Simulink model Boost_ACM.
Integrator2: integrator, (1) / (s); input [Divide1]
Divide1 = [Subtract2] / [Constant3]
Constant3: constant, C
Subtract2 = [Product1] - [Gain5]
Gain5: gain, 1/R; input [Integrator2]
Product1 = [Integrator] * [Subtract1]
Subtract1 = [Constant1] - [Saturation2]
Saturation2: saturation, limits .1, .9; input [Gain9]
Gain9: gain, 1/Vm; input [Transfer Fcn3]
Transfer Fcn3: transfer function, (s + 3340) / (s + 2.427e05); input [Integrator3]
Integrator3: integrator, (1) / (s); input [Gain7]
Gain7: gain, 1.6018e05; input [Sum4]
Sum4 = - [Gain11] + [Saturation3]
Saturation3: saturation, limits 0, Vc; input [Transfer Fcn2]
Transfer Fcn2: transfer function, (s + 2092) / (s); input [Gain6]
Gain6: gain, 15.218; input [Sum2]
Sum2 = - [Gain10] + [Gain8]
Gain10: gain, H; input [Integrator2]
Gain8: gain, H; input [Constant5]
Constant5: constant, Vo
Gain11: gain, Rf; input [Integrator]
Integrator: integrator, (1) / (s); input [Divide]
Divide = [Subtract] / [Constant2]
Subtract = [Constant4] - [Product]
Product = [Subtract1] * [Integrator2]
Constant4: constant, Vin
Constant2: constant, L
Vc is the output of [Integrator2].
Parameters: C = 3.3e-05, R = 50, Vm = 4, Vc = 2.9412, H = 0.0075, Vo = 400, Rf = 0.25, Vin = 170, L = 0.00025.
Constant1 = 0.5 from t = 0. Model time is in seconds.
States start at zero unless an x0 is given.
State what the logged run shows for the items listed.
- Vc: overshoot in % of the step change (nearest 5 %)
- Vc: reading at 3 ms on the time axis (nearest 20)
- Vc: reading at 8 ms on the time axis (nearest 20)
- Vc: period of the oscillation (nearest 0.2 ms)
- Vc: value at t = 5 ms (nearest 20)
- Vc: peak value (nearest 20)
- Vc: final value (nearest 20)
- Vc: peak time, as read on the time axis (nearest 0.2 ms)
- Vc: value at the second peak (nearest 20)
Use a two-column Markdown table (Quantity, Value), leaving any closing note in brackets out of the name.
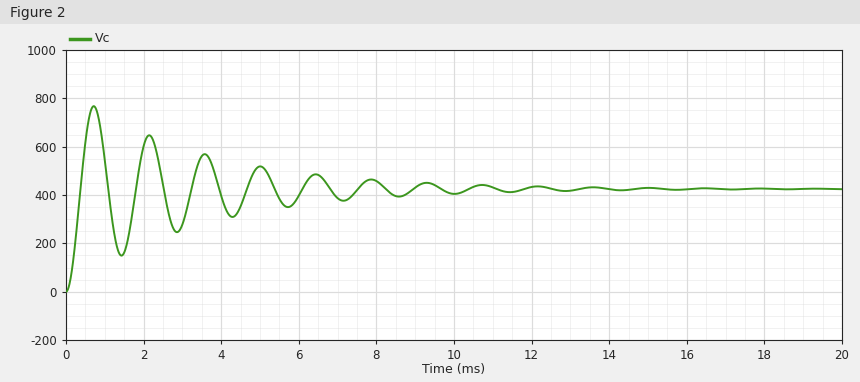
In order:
| Quantity | Value |
|---|---|
| Vc: overshoot in % of the step change | 80 % |
| Vc: reading at 3 ms on the time axis | 280 |
| Vc: reading at 8 ms on the time axis | 460 |
| Vc: period of the oscillation | 1.4 ms |
| Vc: value at t = 5 ms | 520 |
| Vc: peak value | 760 |
| Vc: final value | 420 |
| Vc: peak time, as read on the time axis | 0.8 ms |
| Vc: value at the second peak | 640 |
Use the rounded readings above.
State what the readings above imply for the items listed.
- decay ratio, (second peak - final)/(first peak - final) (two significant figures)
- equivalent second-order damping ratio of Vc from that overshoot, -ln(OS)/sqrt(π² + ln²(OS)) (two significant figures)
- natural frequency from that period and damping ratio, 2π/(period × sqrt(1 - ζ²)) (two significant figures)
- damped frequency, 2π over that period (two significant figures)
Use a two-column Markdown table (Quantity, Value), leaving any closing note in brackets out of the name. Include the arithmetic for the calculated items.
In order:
| Quantity | Value |
|---|---|
| decay ratio, (second peak - final)/(first peak - final) | (640 - 420) / (760 - 420) = 0.65 |
| equivalent second-order damping ratio of Vc from that overshoot, -ln(OS)/sqrt(π² + ln²(OS)) | ln(0.8) = -0.223; 0.223 / sqrt(9.870 + 0.050) = 0.071 |
| natural frequency from that period and damping ratio, 2π/(period × sqrt(1 - ζ²)) | 2π / (1.4 × sqrt(1 - 0.071²)) = 4.5 rad/ms |
| damped frequency, 2π over that period | 2π / 1.4 = 4.5 rad/ms |
